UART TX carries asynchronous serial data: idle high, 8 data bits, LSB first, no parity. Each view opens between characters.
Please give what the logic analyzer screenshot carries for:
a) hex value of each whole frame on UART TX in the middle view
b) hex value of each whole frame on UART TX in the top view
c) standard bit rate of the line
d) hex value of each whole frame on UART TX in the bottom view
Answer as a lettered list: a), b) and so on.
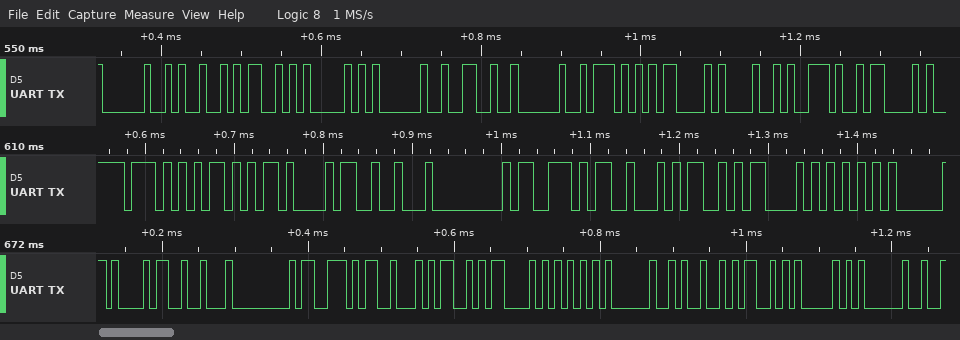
a) 57, AB, A1, 12, 00, 73, 13, 4D, 43, 55
b) 20, 49, 53, 50, 20, 26, 20, 57, 43, 48, 2E, 43
c) 115200 baud
d) A1, 12, 00, 73, 13, 4D, 43, 55, 20, 49, 53, 50, 20
